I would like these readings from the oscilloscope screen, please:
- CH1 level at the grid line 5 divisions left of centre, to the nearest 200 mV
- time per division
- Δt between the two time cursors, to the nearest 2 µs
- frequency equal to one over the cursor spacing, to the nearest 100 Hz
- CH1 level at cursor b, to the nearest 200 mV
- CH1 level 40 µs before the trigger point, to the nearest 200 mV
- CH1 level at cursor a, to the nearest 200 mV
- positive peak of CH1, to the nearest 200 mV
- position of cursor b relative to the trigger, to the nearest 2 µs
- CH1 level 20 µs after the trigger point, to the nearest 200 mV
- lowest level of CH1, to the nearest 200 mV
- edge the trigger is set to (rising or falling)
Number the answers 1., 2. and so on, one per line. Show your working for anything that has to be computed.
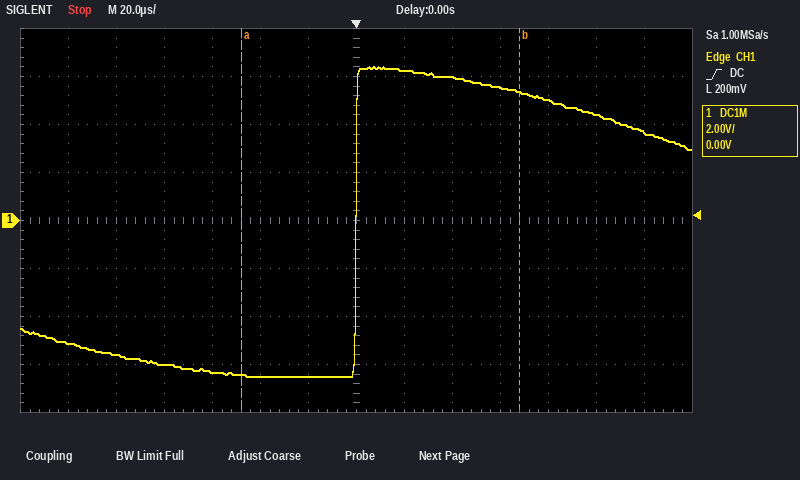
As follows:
1. -5.6 V
2. 20 µs
3. 116 µs
4. 1 / 116 µs ≈ 8.6 kHz
5. 5.4 V
6. -6.4 V
7. -6.4 V
8. 6.4 V
9. +68 µs
10. 6.2 V
11. -6.4 V
12. rising
